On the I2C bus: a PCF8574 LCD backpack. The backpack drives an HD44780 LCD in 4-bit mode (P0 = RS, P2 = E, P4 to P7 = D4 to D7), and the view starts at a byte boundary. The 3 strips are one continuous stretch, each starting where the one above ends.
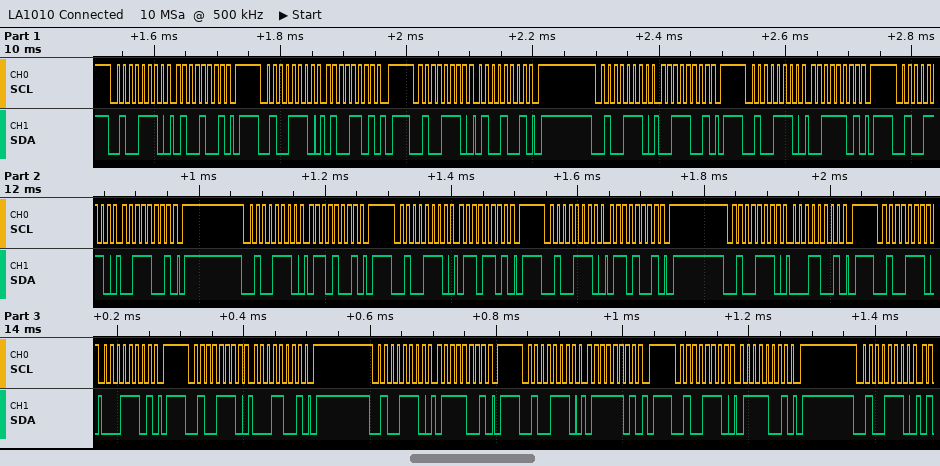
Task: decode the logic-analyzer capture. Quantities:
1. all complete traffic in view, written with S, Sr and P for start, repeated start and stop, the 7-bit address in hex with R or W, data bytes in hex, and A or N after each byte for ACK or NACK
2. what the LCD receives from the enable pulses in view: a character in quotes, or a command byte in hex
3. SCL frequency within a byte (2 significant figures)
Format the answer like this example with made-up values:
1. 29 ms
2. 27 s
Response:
1. S 27W A 49 A P S 27W A 4D A P S 27W A 49 A P S 27W A 39 A P S 27W A 3D A P S 27W A 39 A P S 27W A 69 A P S 27W A 6D A P S 27W A 69 A P S 27W A 19 A P S 27W A 1D A P S 27W A 19 A P S 27W A 79 A P S 27W A 7D A P S 27W A 79 A P S 27W A
2. 'C' 'a'
3. 100 kHz
